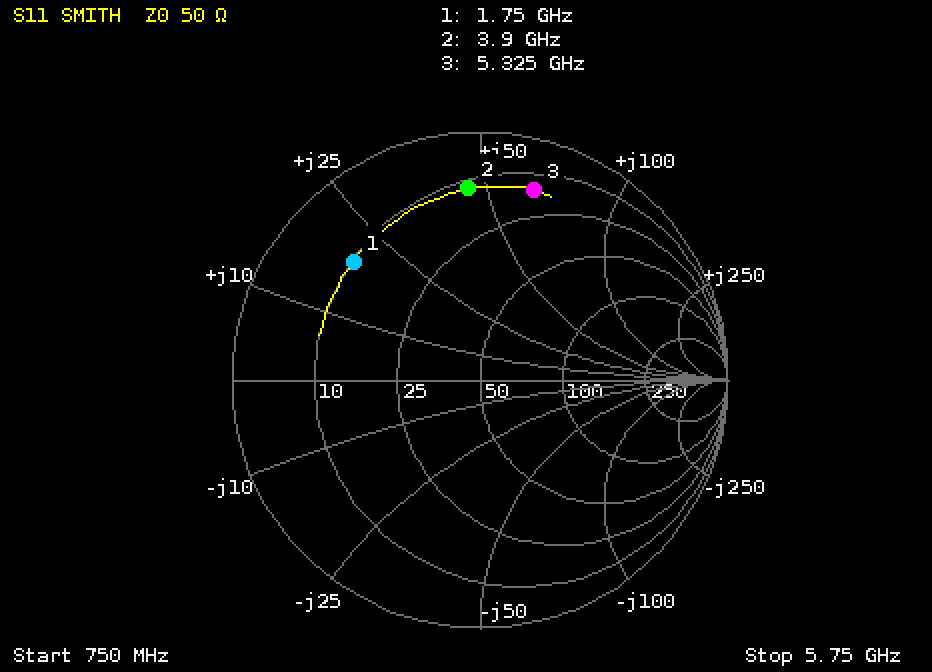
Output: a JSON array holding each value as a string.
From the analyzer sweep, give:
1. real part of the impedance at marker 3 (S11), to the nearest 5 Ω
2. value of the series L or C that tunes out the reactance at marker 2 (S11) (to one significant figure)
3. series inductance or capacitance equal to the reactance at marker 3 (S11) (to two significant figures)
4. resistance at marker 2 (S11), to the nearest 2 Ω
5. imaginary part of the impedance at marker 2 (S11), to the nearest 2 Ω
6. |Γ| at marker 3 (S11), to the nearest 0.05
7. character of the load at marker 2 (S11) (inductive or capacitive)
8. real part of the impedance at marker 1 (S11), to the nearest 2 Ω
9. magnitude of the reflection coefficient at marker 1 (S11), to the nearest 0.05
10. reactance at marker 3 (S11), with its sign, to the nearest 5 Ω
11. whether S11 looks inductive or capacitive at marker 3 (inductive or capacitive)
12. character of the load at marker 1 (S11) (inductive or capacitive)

["15 Ω", "900 fF", "1.9 nH", "12 Ω", "+46 Ω", "0.80", "inductive", "10 Ω", "0.70", "+65 Ω", "inductive", "inductive"]
